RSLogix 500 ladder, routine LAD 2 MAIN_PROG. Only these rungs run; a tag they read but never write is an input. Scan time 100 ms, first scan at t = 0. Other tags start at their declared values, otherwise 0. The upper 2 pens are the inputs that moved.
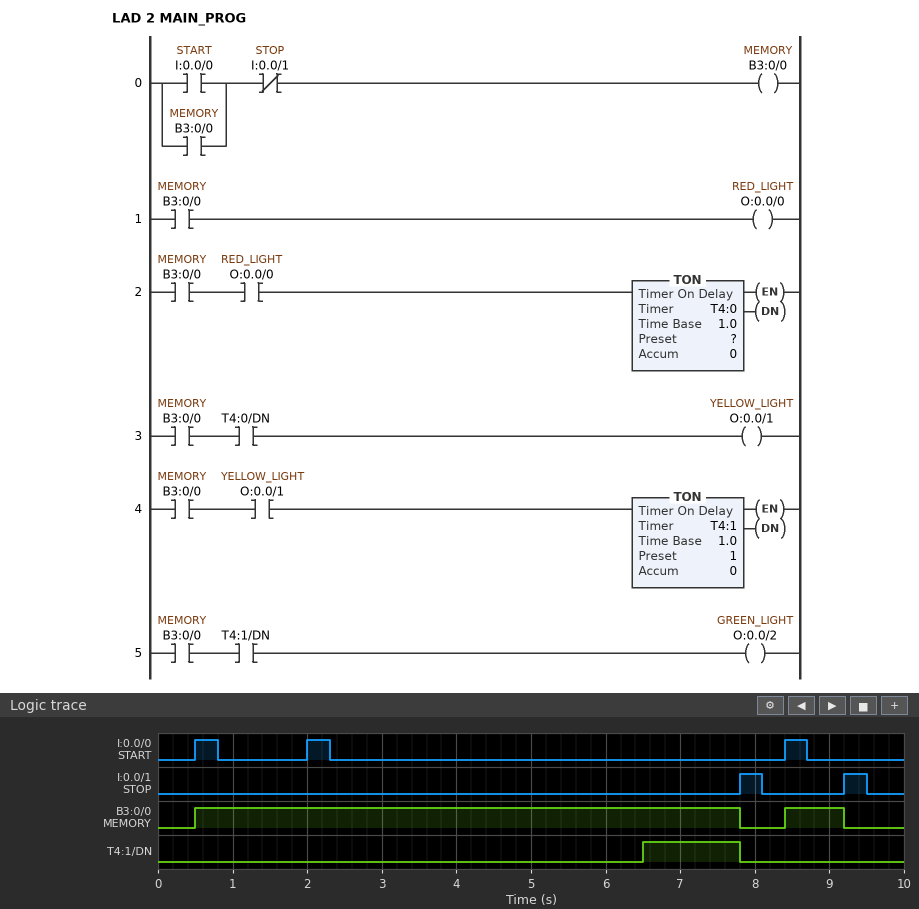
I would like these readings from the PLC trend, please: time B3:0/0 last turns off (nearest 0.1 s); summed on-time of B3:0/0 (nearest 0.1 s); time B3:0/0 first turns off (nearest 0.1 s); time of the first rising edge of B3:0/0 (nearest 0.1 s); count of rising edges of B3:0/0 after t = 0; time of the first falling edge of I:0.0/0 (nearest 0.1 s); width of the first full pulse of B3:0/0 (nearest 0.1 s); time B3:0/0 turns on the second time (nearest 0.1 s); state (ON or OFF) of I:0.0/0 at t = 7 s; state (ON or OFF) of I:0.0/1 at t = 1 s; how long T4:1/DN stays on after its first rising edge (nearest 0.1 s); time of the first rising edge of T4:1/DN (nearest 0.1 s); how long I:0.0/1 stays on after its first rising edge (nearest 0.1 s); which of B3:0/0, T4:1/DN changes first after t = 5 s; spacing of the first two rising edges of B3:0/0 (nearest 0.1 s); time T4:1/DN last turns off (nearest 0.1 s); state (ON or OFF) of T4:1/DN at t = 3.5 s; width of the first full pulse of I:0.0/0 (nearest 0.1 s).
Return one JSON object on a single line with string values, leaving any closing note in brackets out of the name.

{"time B3:0/0 last turns off": "9.2 s", "summed on-time of B3:0/0": "8.1 s", "time B3:0/0 first turns off": "7.8 s", "time of the first rising edge of B3:0/0": "0.5 s", "count of rising edges of B3:0/0 after t = 0": "2", "time of the first falling edge of I:0.0/0": "0.8 s", "width of the first full pulse of B3:0/0": "7.3 s", "time B3:0/0 turns on the second time": "8.4 s", "state (ON or OFF) of I:0.0/0 at t = 7 s": "OFF", "state (ON or OFF) of I:0.0/1 at t = 1 s": "OFF", "how long T4:1/DN stays on after its first rising edge": "1.3 s", "time of the first rising edge of T4:1/DN": "6.5 s", "how long I:0.0/1 stays on after its first rising edge": "0.3 s", "which of B3:0/0, T4:1/DN changes first after t = 5 s": "T4:1/DN", "spacing of the first two rising edges of B3:0/0": "7.9 s", "time T4:1/DN last turns off": "7.8 s", "state (ON or OFF) of T4:1/DN at t = 3.5 s": "OFF", "width of the first full pulse of I:0.0/0": "0.3 s"}
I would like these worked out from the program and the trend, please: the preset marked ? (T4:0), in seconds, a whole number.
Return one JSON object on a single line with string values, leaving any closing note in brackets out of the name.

{"the preset marked ? (T4:0), in seconds, a whole number": "5 s"}
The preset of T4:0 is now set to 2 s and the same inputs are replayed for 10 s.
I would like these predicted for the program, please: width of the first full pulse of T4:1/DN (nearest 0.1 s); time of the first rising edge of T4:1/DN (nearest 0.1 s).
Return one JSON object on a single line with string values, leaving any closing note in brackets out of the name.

{"width of the first full pulse of T4:1/DN": "4.3 s", "time of the first rising edge of T4:1/DN": "3.5 s"}
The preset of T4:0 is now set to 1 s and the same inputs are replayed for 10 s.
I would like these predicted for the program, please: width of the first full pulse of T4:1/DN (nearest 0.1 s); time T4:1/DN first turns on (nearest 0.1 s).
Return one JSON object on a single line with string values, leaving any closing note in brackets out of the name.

{"width of the first full pulse of T4:1/DN": "5.3 s", "time T4:1/DN first turns on": "2.5 s"}
